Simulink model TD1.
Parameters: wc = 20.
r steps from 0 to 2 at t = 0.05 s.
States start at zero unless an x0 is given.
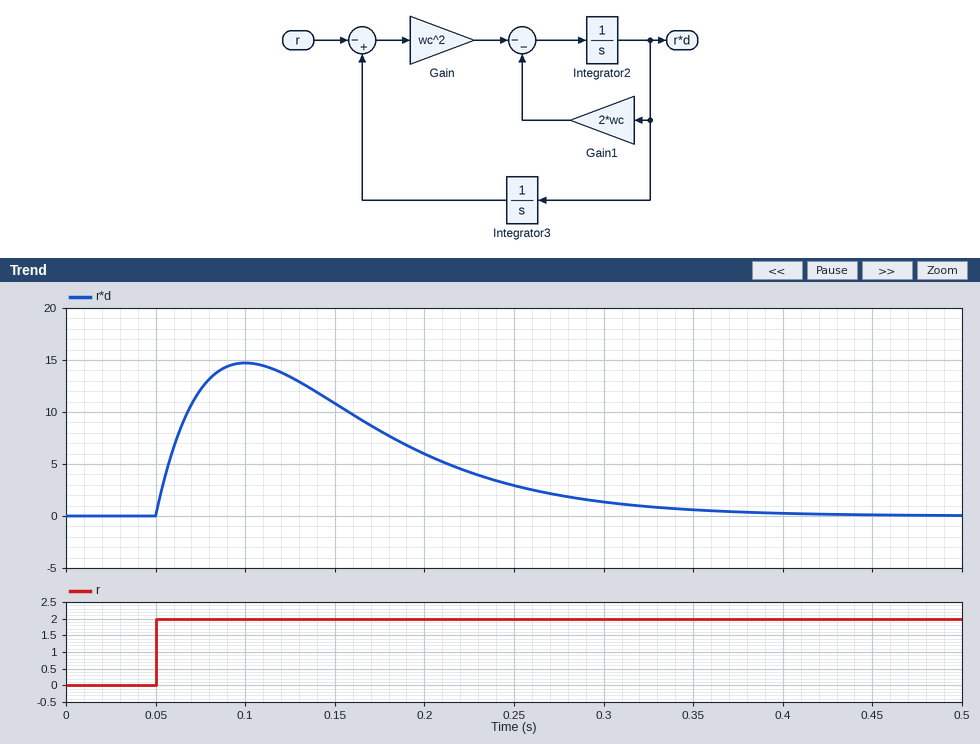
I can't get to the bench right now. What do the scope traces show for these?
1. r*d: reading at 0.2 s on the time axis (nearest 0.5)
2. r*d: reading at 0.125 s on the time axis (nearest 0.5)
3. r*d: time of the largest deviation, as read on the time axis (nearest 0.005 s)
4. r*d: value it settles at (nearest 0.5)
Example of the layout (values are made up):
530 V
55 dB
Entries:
6.0
13.5
0.100 s
0.0
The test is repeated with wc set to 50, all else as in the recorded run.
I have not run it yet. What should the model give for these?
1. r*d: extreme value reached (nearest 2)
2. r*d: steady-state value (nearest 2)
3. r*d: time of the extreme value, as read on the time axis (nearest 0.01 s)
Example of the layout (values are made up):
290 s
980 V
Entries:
36
0
0.07 s
